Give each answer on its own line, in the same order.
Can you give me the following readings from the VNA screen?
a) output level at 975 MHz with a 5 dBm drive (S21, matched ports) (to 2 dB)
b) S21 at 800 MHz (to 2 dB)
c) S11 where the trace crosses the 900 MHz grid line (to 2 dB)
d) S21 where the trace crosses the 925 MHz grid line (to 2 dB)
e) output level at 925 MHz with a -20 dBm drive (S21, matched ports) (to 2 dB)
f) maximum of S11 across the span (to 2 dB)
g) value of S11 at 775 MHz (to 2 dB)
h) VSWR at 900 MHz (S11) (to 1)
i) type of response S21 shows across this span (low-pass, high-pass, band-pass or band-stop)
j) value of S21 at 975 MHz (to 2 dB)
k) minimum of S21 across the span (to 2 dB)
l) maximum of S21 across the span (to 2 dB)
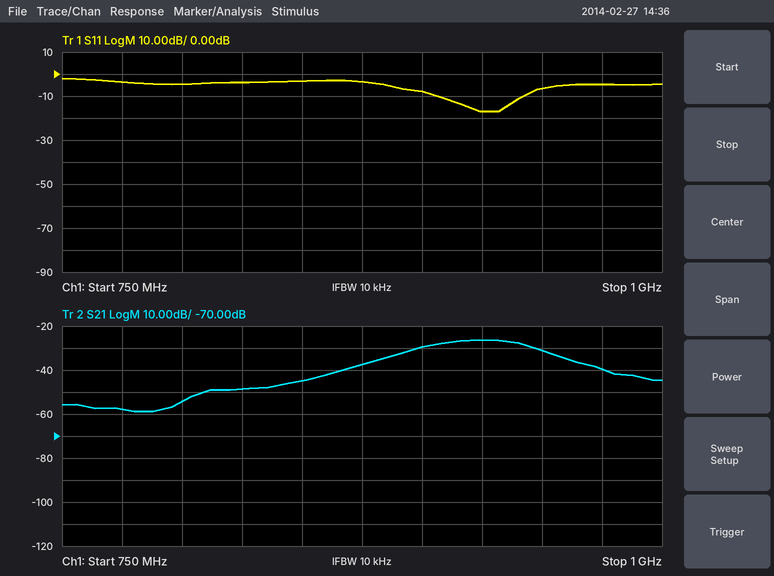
-34 dBm
-54 dB
-8 dB
-26 dB
-46 dBm
-2 dB
-4 dB
2
band-pass
-40 dB
-58 dB
-26 dB
